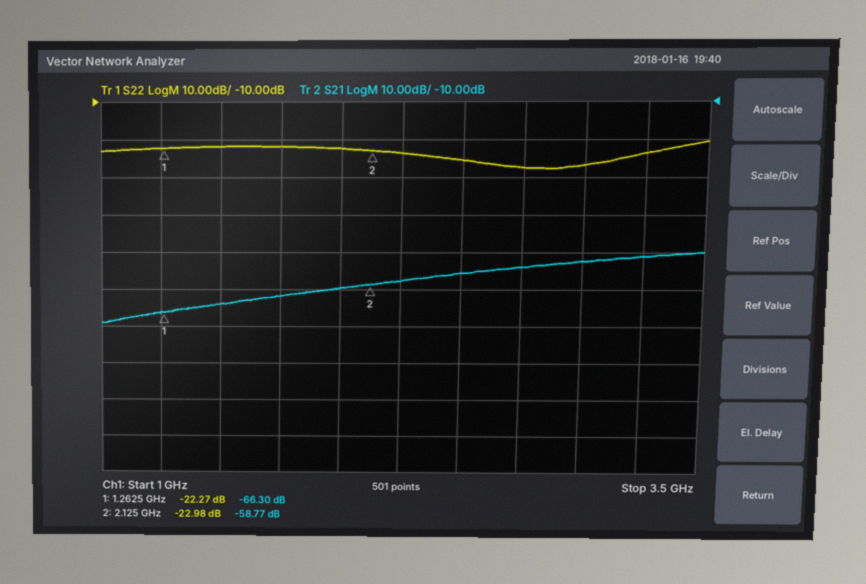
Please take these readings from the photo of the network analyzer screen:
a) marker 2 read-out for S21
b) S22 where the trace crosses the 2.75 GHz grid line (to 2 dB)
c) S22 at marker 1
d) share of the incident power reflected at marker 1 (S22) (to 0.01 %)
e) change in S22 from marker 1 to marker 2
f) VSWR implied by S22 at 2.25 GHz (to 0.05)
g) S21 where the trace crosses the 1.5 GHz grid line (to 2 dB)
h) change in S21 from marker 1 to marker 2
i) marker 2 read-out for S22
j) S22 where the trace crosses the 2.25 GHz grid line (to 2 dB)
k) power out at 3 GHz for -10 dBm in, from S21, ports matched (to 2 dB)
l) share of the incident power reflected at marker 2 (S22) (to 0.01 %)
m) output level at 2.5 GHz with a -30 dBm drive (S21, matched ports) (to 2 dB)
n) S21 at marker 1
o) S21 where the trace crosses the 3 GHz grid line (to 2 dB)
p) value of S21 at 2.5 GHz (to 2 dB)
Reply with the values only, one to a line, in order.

-58.77 dB
-28 dB
-22.27 dB
0.59 %
-0.71 dB
1.15
-64 dB
7.53 dB
-22.98 dB
-24 dB
-62 dBm
0.50 %
-86 dBm
-66.30 dB
-52 dB
-56 dB
